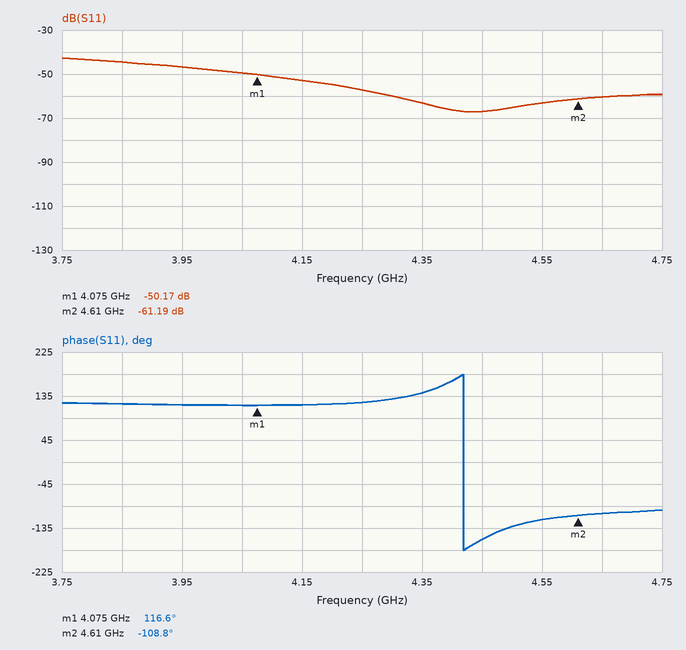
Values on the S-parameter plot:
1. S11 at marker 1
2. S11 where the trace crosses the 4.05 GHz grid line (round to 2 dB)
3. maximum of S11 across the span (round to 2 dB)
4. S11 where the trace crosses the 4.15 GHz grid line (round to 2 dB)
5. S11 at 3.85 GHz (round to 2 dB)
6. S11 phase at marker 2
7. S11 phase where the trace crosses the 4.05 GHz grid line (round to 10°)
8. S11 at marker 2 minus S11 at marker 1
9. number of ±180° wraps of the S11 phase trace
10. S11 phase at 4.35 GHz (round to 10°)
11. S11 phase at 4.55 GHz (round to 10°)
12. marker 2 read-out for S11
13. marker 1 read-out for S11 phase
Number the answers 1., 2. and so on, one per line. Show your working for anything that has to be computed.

1. -50.17 dB
2. -50 dB
3. -42 dB
4. -52 dB
5. -44 dB
6. -108.8°
7. 120°
8. -61.19 − (-50.17) = -11.02 dB
9. 1
10. 140°
11. -120°
12. -61.19 dB
13. 116.6°
